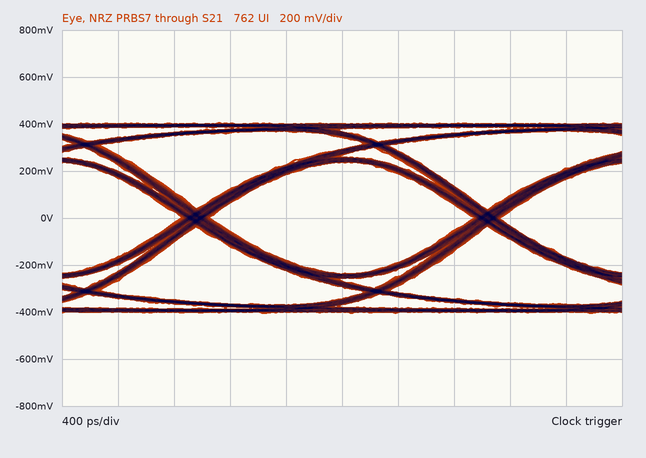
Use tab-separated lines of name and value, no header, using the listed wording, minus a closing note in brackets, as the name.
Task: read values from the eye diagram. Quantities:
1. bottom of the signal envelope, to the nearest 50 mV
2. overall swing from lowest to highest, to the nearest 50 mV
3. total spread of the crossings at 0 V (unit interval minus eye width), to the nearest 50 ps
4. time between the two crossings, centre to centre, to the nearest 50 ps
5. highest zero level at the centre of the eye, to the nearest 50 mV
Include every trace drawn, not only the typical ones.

bottom of the signal envelope, to the nearest 50 mV	-400 mV
overall swing from lowest to highest, to the nearest 50 mV	800 mV
total spread of the crossings at 0 V (unit interval minus eye width), to the nearest 50 ps	200 ps
time between the two crossings, centre to centre, to the nearest 50 ps	2.10 ns
highest zero level at the centre of the eye, to the nearest 50 mV	-250 mV
